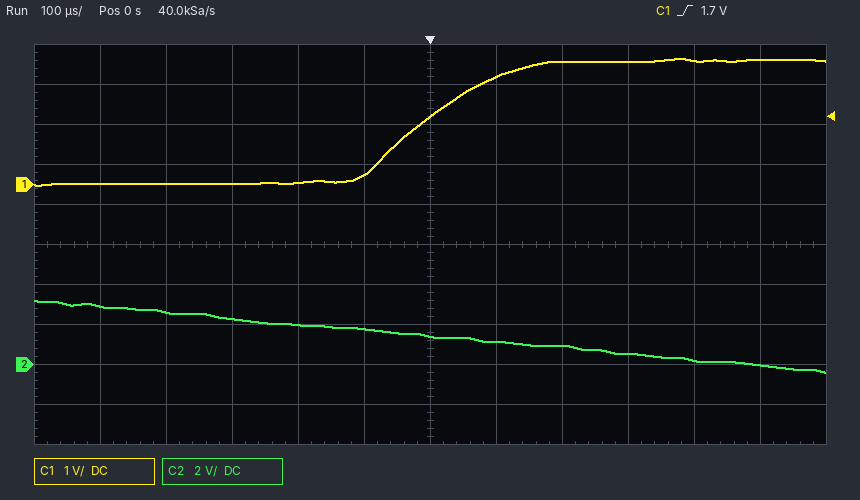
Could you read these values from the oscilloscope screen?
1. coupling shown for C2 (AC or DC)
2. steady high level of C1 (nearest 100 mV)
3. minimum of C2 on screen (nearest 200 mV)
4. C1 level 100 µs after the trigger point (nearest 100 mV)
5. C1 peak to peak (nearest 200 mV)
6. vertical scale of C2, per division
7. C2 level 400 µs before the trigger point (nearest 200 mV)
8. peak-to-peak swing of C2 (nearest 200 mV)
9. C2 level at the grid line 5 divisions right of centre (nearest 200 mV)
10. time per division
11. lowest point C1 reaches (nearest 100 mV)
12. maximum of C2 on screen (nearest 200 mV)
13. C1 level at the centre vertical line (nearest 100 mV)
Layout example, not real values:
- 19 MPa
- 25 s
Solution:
- DC
- 3.1 V
- -400 mV
- 2.7 V
- 3.2 V
- 2 V
- 2.6 V
- 3.6 V
- 0.0 V
- 100 µs
- 0.0 V
- 3.2 V
- 1.7 V
